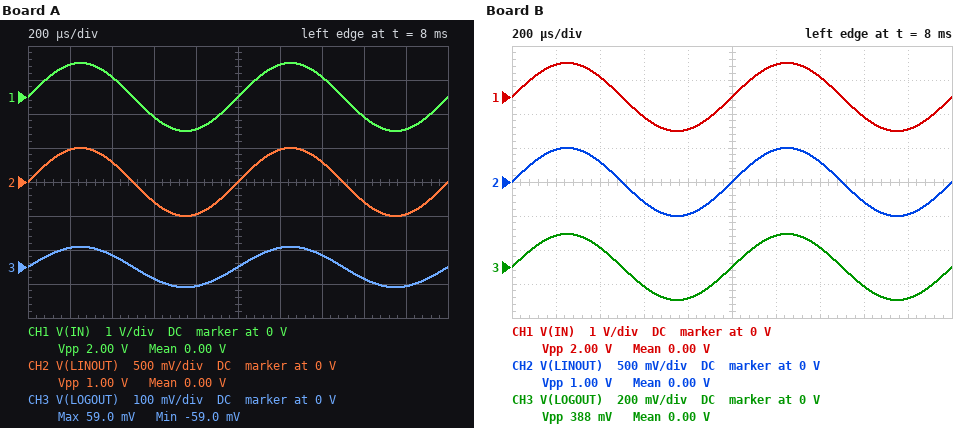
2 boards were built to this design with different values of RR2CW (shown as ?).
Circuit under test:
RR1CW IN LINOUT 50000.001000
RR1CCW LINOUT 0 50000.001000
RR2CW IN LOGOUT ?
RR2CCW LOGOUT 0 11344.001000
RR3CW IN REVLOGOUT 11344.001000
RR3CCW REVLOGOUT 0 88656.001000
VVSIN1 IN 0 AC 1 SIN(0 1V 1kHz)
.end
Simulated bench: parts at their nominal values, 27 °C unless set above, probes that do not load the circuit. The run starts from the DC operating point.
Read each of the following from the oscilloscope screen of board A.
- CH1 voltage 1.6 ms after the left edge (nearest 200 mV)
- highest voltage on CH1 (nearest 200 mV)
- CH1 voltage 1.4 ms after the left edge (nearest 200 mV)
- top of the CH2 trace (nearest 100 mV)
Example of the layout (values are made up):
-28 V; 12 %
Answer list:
-600 mV; 1.0 V; 600 mV; 500 mV
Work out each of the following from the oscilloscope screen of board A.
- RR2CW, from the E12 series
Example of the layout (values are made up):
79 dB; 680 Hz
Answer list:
180 kΩ
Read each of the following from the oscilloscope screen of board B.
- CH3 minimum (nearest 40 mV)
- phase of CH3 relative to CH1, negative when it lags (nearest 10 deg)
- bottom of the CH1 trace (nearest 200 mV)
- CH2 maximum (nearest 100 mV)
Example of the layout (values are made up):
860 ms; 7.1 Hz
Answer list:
-200 mV; 0 deg; -1.0 V; 500 mV
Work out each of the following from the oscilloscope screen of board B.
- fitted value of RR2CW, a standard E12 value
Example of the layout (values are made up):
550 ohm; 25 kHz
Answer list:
47 kΩ
